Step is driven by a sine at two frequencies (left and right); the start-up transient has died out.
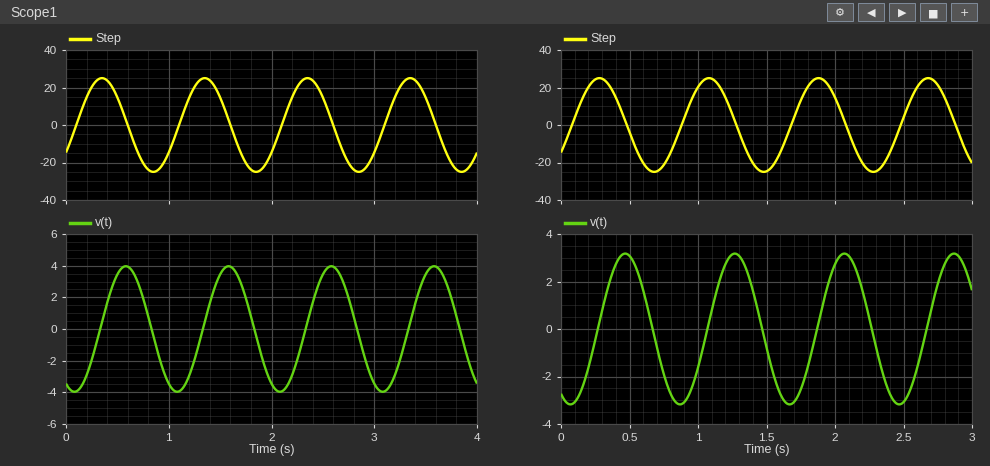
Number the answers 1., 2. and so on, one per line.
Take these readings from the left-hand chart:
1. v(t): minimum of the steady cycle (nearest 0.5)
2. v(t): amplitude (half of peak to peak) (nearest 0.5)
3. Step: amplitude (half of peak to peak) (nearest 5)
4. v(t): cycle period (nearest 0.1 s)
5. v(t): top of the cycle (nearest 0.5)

1. -4.0
2. 4.0
3. 25
4. 1.0 s
5. 4.0
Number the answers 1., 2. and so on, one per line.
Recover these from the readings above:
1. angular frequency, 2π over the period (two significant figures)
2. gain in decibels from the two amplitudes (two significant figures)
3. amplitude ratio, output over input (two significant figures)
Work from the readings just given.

1. 6.3 rad/s
2. -16 dB
3. 0.16
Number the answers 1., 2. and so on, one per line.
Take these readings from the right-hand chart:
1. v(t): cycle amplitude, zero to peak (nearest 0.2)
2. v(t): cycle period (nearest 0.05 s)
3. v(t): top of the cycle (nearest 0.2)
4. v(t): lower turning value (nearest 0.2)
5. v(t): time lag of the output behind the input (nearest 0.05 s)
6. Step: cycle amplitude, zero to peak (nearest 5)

1. 3.2
2. 0.80 s
3. 3.2
4. -3.2
5. 0.20 s
6. 25
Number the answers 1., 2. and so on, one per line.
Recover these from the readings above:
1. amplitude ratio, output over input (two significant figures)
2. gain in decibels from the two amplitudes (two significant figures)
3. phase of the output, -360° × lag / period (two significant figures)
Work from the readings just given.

1. 0.13
2. -18 dB
3. -90°
